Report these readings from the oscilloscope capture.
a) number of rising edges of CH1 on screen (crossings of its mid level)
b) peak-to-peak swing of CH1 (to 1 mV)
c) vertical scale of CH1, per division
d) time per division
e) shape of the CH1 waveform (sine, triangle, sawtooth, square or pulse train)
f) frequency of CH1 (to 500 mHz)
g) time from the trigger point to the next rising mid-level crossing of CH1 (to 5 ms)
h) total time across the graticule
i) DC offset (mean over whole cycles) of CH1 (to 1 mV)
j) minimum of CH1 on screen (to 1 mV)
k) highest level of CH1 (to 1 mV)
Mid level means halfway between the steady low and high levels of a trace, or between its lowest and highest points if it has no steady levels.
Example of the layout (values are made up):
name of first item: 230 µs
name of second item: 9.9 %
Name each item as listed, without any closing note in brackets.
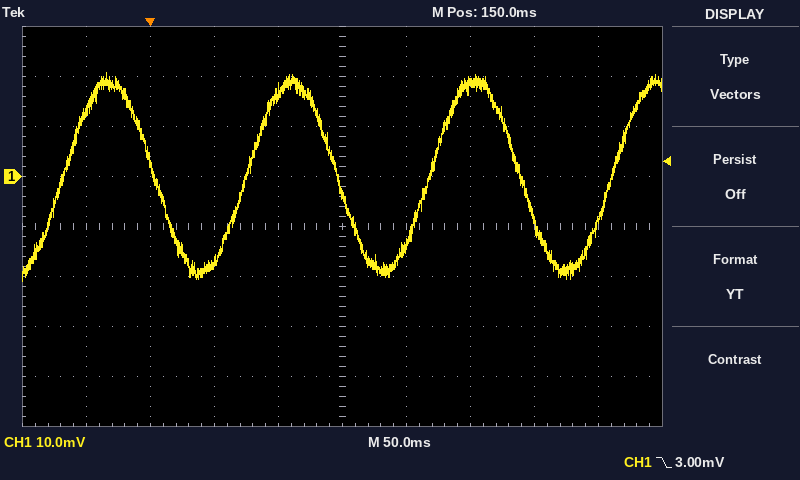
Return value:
number of rising edges of CH1 on screen: 4
peak-to-peak swing of CH1: 42 mV
vertical scale of CH1, per division: 10 mV
time per division: 50 ms
shape of the CH1 waveform: sine
frequency of CH1: 7.0 Hz
time from the trigger point to the next rising mid-level crossing of CH1: 75 ms
total time across the graticule: 500 ms
DC offset (mean over whole cycles) of CH1: 0 mV
minimum of CH1 on screen: -21 mV
highest level of CH1: 21 mV
